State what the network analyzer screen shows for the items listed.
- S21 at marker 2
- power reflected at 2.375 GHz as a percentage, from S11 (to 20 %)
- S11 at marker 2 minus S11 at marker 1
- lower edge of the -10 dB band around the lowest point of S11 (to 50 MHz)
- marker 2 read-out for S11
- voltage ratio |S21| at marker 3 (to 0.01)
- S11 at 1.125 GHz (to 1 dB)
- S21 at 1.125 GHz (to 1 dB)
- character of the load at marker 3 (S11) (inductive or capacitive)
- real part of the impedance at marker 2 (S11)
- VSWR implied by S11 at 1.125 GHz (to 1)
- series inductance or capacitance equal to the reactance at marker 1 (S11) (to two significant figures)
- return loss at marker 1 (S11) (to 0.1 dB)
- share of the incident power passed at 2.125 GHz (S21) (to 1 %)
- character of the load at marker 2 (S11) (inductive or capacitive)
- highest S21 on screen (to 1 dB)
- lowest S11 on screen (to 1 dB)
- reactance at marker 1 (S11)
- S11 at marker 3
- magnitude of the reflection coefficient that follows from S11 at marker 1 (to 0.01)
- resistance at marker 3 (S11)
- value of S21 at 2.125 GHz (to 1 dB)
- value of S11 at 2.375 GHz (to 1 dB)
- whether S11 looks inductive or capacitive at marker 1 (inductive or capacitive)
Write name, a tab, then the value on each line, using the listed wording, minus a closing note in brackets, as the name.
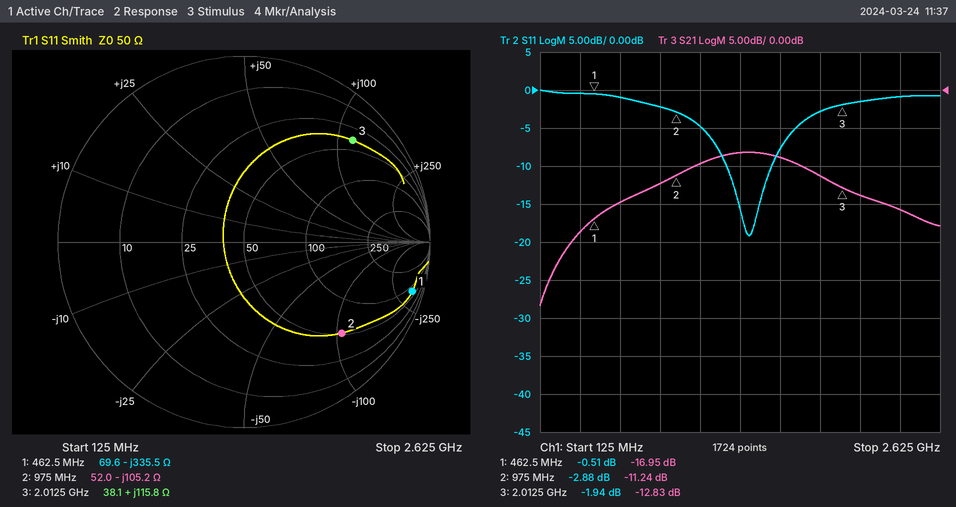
S21 at marker 2	-11.24 dB
power reflected at 2.375 GHz as a percentage, from S11	80 %
S11 at marker 2 minus S11 at marker 1	-2.37 dB
lower edge of the -10 dB band around the lowest point of S11	1.30 GHz
marker 2 read-out for S11	-2.88 dB
voltage ratio |S21| at marker 3	0.23
S11 at 1.125 GHz	-5 dB
S21 at 1.125 GHz	-10 dB
character of the load at marker 3 (S11)	inductive
real part of the impedance at marker 2	52.0 Ω
VSWR implied by S11 at 1.125 GHz	4
series inductance or capacitance equal to the reactance at marker 1 (S11)	1.0 pF
return loss at marker 1 (S11)	0.5 dB
share of the incident power passed at 2.125 GHz (S21)	4 %
character of the load at marker 2 (S11)	capacitive
highest S21 on screen	-8 dB
lowest S11 on screen	-19 dB
reactance at marker 1	-335.5 Ω
S11 at marker 3	-1.94 dB
magnitude of the reflection coefficient that follows from S11 at marker 1	0.94
resistance at marker 3	38.1 Ω
value of S21 at 2.125 GHz	-14 dB
value of S11 at 2.375 GHz	-1 dB
whether S11 looks inductive or capacitive at marker 1	capacitive
